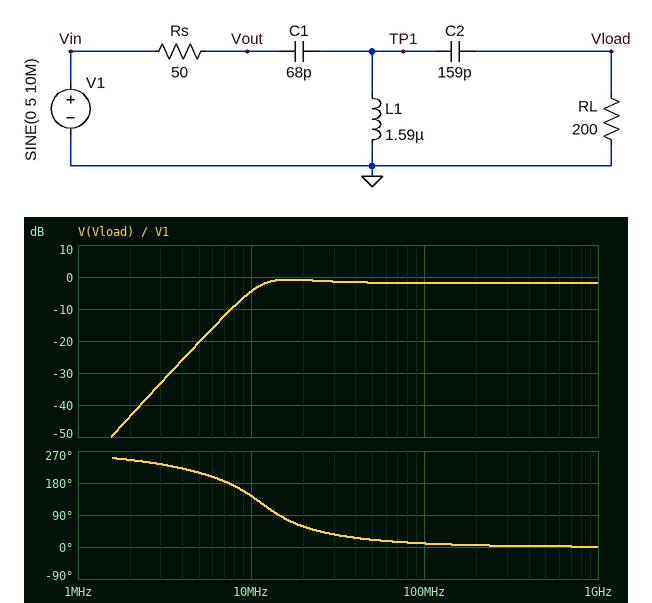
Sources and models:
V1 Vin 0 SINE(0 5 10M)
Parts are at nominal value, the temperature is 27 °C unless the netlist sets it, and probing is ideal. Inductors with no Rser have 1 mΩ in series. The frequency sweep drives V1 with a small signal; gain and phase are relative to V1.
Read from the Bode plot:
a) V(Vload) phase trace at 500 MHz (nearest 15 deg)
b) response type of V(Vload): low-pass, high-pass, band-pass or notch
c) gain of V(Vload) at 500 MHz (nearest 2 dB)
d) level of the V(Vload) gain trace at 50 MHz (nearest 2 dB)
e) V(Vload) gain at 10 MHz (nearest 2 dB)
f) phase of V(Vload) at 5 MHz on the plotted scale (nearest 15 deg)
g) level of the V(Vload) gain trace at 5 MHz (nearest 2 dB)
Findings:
0 deg
high-pass
-2 dB
-2 dB
-4 dB
210 deg
-20 dB
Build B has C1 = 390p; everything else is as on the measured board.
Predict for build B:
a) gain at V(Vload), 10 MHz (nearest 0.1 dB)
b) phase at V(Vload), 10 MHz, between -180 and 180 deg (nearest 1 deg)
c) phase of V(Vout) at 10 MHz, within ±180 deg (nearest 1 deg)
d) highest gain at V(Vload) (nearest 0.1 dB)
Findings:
-1.3 dB
59 deg
19 deg
-1.0 dB
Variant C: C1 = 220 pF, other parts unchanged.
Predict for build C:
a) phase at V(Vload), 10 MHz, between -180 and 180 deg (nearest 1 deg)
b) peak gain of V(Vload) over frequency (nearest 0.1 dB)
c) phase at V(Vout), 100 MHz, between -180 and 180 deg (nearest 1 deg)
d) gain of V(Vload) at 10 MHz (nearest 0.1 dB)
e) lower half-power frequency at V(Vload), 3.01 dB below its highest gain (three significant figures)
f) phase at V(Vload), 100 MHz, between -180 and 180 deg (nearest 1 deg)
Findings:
75 deg
-0.1 dB
1 deg
-0.3 dB
6.23 MHz
6 deg
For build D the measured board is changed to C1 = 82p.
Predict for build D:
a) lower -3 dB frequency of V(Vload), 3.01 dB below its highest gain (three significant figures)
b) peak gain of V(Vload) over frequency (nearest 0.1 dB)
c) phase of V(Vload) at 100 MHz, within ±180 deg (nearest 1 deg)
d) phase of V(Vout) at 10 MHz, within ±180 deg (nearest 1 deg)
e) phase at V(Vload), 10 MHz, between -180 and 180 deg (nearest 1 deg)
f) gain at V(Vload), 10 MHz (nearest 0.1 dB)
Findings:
9.53 MHz
-0.5 dB
9 deg
-19 deg
133 deg
-2.8 dB
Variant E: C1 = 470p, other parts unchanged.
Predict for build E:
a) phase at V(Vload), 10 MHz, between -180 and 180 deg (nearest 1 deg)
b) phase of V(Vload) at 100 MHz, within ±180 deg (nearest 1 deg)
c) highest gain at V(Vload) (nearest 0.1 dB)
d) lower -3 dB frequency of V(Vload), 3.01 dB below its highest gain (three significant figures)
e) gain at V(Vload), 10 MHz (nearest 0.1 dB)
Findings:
57 deg
5 deg
-1.4 dB
4.69 MHz
-1.6 dB
